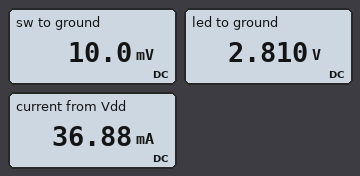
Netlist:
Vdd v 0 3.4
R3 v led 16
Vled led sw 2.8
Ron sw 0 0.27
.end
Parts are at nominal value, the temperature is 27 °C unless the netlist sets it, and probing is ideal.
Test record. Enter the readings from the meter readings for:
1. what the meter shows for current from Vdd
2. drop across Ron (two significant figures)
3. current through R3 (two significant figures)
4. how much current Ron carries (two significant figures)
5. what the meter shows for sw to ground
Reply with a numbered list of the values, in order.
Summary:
1. 36.88 mA
2. 10 mV
3. 37 mA
4. 37 mA
5. 10.0 mV
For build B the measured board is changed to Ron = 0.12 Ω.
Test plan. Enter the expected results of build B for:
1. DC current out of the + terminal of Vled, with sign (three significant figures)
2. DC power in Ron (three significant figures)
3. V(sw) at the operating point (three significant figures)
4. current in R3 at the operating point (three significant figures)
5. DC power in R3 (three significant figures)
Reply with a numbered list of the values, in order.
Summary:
1. -37.2 mA
2. 166 µW
3. 4.47 mV
4. 37.2 mA
5. 22.2 mW
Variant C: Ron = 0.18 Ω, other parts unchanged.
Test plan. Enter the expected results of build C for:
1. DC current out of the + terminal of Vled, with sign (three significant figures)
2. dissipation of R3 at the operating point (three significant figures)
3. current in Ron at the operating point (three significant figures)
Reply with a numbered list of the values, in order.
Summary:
1. -37.1 mA
2. 22.0 mW
3. 37.1 mA
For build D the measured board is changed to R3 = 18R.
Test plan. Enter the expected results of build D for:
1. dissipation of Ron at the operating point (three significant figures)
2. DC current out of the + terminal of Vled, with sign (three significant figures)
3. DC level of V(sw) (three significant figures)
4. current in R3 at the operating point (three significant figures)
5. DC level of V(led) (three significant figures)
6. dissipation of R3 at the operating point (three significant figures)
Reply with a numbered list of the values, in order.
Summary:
1. 291 µW
2. -32.8 mA
3. 8.87 mV
4. 32.8 mA
5. 2.81 V
6. 19.4 mW
